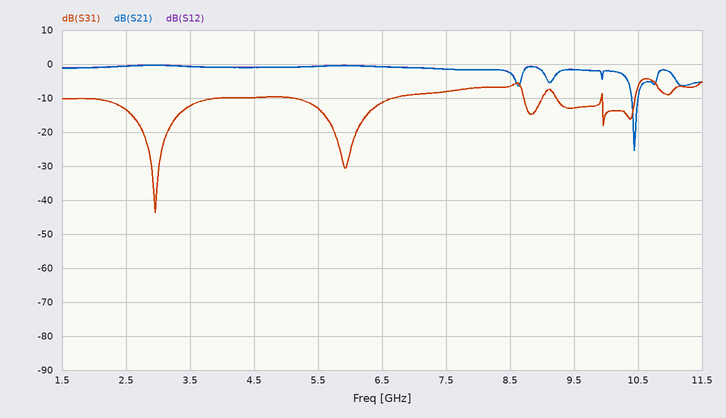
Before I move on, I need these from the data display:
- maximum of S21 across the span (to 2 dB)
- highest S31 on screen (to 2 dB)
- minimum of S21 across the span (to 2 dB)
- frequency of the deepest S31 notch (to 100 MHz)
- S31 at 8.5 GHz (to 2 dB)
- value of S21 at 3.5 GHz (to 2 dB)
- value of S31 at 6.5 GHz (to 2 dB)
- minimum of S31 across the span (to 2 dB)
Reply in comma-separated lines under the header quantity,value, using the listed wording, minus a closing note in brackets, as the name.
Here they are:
quantity,value
maximum of S21 across the span,0 dB
highest S31 on screen,-4 dB
minimum of S21 across the span,-26 dB
frequency of the deepest S31 notch,3.0 GHz
S31 at 8.5 GHz,-6 dB
value of S21 at 3.5 GHz,0 dB
value of S31 at 6.5 GHz,-12 dB
minimum of S31 across the span,-44 dB
